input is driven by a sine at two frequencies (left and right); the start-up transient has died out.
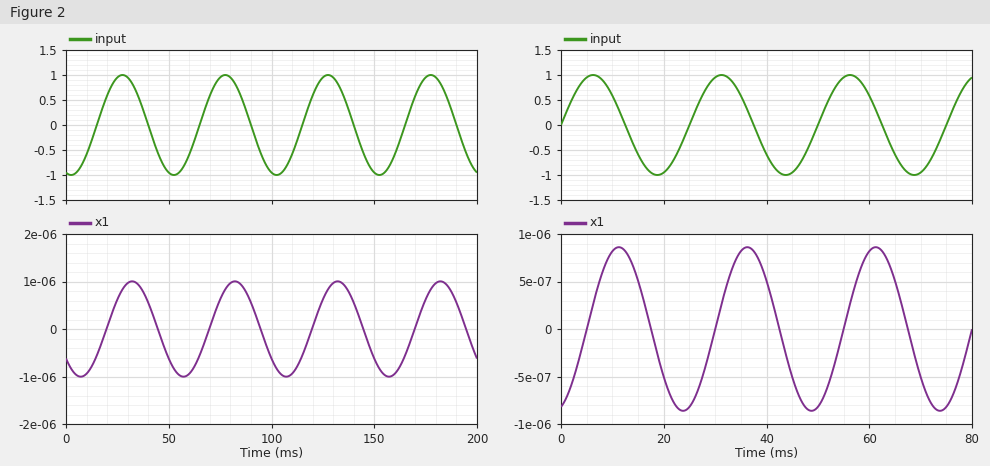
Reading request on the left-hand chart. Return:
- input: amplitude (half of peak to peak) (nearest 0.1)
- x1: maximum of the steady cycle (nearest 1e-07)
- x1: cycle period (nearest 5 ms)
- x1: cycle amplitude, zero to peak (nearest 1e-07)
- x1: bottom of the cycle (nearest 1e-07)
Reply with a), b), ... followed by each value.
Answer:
a) 1.0
b) 0.0000010
c) 50 ms
d) 0.0000010
e) -0.0000010
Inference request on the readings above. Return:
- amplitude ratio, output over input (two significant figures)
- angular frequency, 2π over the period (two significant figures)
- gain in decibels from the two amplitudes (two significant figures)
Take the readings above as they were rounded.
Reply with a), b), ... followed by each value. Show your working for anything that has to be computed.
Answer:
a) 1e-06 / 1 = 0.0000010
b) 2π / 50 = 0.13 rad/ms
c) 20 log10(1e-06 / 1) = -120 dB
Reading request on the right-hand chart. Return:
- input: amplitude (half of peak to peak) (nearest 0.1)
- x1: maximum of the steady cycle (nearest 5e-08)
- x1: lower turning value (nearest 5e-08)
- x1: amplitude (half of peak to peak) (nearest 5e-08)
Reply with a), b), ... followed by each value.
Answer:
a) 1.0
b) 0.00000085
c) -0.00000085
d) 0.00000085
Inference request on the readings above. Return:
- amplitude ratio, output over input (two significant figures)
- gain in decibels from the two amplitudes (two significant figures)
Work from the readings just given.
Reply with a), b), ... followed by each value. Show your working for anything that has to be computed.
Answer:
a) 8.5e-07 / 1 = 0.00000085
b) 20 log10(8.5e-07 / 1) = -120 dB
